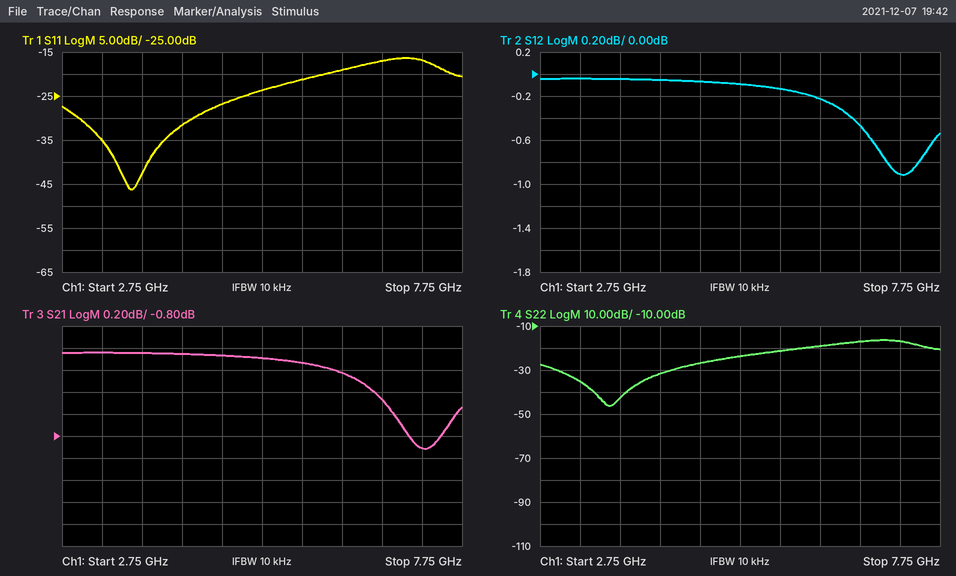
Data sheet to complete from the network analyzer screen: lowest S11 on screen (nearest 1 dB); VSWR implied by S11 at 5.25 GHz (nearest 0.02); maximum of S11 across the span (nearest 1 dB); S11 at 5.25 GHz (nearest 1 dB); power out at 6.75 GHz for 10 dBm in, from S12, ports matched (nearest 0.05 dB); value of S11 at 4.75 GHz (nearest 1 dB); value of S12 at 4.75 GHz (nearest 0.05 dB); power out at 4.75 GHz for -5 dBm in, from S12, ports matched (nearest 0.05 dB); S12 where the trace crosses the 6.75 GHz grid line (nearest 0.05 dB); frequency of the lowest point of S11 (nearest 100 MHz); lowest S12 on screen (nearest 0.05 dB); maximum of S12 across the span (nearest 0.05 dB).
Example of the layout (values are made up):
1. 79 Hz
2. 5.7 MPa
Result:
1. -46 dB
2. 1.14
3. -16 dB
4. -24 dB
5. 9.55 dBm
6. -27 dB
7. -0.05 dB
8. -5.05 dBm
9. -0.45 dB
10. 3.6 GHz
11. -0.90 dB
12. -0.05 dB
